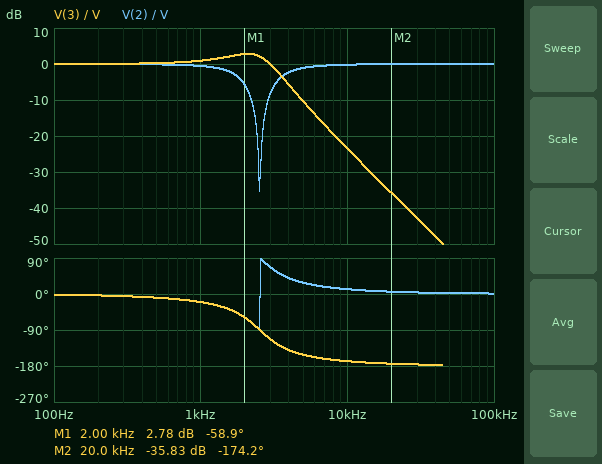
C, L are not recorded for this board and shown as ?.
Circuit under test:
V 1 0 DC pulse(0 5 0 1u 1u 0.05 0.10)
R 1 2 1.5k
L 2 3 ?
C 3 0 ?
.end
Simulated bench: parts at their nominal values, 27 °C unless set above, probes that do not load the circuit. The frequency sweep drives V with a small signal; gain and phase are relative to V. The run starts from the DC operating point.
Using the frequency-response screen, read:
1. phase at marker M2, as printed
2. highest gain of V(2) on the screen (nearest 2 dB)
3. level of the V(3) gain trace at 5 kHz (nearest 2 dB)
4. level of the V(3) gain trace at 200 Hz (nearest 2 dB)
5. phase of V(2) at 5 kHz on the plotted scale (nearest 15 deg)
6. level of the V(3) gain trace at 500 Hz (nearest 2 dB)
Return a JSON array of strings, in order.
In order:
["-174.2 deg", "0 dB", "-10 dB", "0 dB", "30 deg", "0 dB"]
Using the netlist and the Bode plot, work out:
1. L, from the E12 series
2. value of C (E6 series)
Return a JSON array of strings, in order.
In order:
["120 mH", "33 nF"]
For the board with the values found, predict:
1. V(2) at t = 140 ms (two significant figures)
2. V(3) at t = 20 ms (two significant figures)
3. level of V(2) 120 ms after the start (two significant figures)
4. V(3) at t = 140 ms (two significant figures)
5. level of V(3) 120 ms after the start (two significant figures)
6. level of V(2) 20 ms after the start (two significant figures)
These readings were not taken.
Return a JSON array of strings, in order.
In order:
["5.0 V", "5.0 V", "5.0 V", "5.0 V", "5.0 V", "5.0 V"]
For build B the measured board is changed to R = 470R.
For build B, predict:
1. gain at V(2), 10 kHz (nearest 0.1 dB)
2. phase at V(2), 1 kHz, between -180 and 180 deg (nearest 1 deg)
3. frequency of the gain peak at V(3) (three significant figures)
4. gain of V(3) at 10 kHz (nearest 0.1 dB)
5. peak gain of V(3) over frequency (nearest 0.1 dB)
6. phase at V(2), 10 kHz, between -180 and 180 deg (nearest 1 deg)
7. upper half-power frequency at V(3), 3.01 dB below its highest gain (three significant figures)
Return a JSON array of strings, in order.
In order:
["0 dB", "-7 deg", "2.49 kHz", "-23.3 dB", "12.2 dB", "4 deg", "2.79 kHz"]
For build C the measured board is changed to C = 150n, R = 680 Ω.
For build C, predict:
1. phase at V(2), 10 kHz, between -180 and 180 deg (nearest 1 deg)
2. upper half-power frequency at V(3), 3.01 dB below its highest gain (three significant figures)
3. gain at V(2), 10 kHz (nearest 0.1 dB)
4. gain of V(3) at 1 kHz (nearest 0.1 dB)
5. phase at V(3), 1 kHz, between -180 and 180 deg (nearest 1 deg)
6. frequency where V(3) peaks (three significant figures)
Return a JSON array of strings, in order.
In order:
["5 deg", "1.41 kHz", "0 dB", "3.1 dB", "-66 deg", "1.00 kHz"]
